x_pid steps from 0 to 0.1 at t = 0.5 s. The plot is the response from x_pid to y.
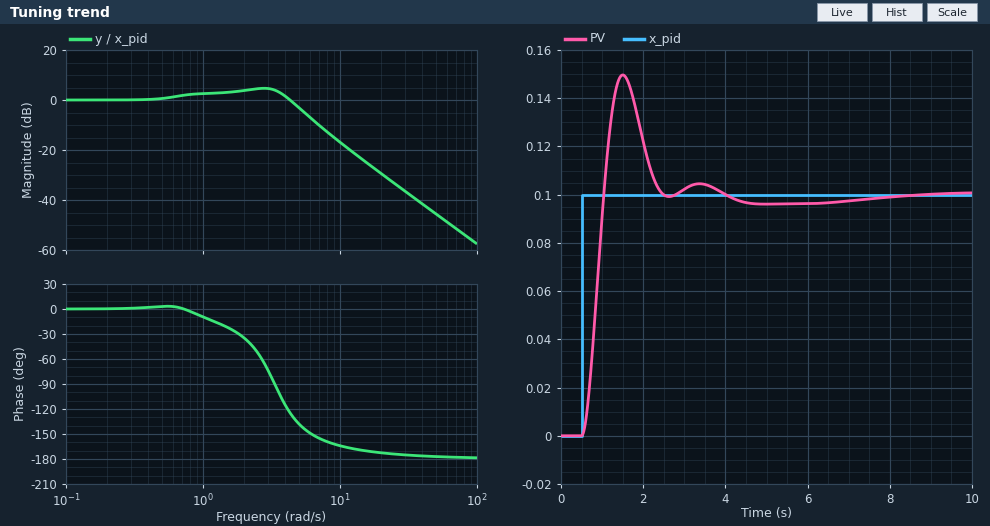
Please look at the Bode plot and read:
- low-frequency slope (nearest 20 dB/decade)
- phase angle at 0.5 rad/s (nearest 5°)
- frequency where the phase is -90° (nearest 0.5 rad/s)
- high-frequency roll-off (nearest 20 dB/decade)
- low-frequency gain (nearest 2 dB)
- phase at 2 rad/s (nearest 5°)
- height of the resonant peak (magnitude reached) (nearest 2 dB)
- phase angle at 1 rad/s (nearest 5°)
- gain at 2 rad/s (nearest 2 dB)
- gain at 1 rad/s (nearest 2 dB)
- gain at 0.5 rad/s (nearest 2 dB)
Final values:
0 dB/decade
5°
3.5 rad/s
-40 dB/decade
0 dB
-35°
4 dB
-10°
4 dB
2 dB
0 dB
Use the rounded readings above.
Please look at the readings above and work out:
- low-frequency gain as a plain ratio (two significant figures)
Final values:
1.0
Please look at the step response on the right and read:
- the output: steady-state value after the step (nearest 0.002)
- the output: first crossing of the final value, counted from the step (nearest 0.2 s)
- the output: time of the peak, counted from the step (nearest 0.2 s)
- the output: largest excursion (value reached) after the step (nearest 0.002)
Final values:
0.100
0.6 s
1.0 s
0.150
